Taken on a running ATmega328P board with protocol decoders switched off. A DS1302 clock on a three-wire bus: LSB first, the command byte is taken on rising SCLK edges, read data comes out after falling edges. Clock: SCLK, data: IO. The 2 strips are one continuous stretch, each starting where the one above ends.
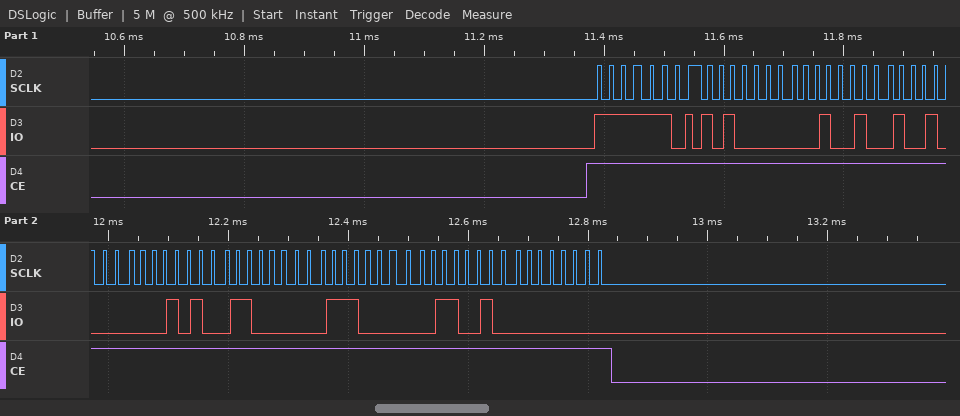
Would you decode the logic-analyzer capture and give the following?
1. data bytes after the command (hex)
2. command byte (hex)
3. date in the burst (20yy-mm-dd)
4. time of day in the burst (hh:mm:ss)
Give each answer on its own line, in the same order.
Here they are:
05 24 09 28 03 07 26 00
0xBF
2026-03-28
09:24:05
